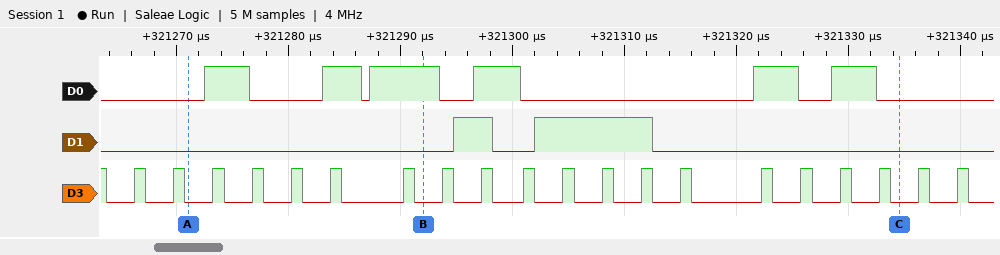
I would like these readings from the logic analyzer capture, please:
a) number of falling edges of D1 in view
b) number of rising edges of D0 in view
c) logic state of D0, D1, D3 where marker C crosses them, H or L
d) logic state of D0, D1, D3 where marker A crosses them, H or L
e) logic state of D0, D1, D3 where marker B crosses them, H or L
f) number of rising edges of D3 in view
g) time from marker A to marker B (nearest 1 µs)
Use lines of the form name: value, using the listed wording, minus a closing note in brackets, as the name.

number of falling edges of D1 in view: 2
number of rising edges of D0 in view: 6
logic state of D0, D1, D3 where marker C crosses them, H or L: D0=L, D1=L, D3=L
logic state of D0, D1, D3 where marker A crosses them, H or L: D0=L, D1=L, D3=L
logic state of D0, D1, D3 where marker B crosses them, H or L: D0=H, D1=L, D3=L
number of rising edges of D3 in view: 20
time from marker A to marker B: 21 µs
